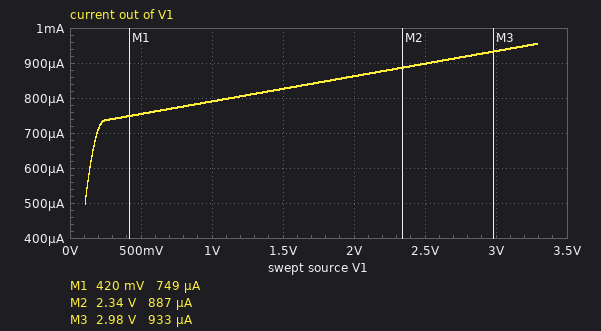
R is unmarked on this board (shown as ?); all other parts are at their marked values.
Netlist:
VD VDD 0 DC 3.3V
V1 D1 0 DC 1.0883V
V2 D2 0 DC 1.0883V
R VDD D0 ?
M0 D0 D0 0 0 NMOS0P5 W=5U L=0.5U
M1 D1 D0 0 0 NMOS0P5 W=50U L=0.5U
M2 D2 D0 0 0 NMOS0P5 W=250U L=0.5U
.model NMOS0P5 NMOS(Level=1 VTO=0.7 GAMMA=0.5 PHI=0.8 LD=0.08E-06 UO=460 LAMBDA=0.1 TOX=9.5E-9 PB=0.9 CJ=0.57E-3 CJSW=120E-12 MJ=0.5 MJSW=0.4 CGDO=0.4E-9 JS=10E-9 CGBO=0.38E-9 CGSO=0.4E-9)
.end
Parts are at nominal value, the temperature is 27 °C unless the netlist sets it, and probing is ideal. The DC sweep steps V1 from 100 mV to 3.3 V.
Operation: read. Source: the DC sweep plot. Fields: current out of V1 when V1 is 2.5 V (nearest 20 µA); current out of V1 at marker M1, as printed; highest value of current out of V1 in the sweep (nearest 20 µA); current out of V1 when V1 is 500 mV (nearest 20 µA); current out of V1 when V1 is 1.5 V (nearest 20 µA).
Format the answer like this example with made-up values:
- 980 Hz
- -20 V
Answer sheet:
- 900 µA
- 749 µA
- 960 µA
- 760 µA
- 820 µA
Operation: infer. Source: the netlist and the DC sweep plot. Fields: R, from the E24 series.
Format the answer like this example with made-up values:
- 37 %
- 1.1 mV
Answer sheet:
- 30 kΩ
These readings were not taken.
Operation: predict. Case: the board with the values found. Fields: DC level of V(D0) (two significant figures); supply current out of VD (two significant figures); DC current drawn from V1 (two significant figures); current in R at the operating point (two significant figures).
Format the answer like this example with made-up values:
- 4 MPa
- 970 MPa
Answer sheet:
- 940 mV
- 79 µA
- 800 µA
- 79 µA
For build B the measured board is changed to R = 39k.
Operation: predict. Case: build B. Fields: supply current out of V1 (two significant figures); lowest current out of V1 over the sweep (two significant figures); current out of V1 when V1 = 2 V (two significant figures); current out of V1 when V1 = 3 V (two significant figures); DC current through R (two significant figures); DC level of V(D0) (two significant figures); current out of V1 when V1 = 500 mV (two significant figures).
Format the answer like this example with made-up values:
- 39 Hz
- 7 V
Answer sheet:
- 620 µA
- 410 µA
- 670 µA
- 730 µA
- 61 µA
- 910 mV
- 590 µA
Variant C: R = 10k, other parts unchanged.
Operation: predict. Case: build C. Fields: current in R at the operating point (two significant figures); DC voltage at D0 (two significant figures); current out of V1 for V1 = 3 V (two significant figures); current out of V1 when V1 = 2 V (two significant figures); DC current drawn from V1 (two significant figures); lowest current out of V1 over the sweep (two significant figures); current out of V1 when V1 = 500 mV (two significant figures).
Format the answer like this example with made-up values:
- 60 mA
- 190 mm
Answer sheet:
- 220 µA
- 1.1 V
- 2.6 mA
- 2.4 mA
- 2.2 mA
- 870 µA
- 2.1 mA
